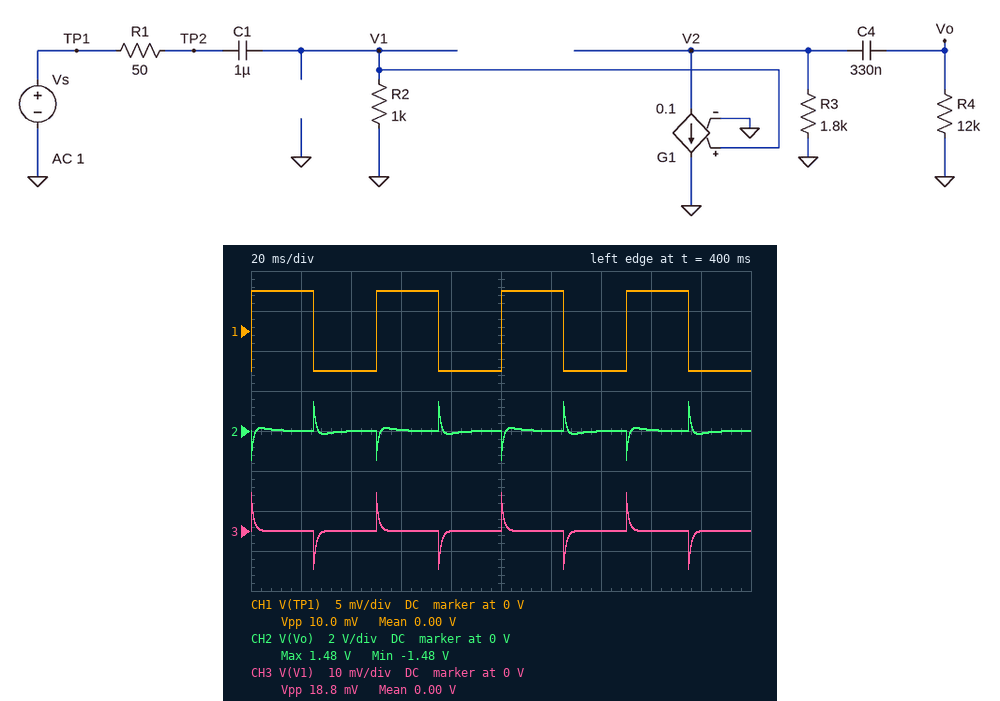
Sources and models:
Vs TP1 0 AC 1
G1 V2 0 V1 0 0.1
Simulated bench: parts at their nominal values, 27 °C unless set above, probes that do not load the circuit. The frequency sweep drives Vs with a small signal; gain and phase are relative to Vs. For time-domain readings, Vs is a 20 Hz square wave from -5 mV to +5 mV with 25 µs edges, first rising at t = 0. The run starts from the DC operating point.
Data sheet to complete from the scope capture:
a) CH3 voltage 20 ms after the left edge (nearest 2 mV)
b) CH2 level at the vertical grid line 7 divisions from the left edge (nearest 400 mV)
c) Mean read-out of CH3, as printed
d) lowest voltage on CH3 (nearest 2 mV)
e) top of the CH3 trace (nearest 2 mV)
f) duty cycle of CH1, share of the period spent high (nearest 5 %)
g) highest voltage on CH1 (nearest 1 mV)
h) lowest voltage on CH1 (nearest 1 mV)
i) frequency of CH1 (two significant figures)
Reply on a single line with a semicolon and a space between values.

0 V; 0 V; 0.00 V; -10 mV; 10 mV; 50 %; 5 mV; -5 mV; 20 Hz
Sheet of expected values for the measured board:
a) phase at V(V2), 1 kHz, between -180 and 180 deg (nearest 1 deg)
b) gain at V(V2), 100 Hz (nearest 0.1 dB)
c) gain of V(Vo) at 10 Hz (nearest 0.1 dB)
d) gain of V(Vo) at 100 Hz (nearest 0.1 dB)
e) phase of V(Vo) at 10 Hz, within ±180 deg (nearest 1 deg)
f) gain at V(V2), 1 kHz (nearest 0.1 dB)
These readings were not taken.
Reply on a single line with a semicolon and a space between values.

-172 deg; 38.4 dB; 8.6 dB; 37.8 dB; -20 deg; 43.4 dB
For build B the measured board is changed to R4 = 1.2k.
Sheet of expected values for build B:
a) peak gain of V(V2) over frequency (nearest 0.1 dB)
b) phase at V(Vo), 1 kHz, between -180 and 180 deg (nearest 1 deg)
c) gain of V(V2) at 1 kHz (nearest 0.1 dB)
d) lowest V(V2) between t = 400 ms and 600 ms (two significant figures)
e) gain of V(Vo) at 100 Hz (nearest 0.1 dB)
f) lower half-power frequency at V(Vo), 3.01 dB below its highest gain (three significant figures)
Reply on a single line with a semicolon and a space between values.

39.6 dB; -162 deg; 37.2 dB; -750 mV; 26.0 dB; 243 Hz
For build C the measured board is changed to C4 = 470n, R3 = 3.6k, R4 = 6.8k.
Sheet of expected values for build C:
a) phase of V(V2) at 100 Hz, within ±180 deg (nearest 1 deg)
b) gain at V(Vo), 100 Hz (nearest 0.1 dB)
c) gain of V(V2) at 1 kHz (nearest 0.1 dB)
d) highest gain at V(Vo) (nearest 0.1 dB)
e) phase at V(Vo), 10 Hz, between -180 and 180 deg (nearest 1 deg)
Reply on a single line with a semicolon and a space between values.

-132 deg; 41.4 dB; 46.9 dB; 47.0 dB; -21 deg
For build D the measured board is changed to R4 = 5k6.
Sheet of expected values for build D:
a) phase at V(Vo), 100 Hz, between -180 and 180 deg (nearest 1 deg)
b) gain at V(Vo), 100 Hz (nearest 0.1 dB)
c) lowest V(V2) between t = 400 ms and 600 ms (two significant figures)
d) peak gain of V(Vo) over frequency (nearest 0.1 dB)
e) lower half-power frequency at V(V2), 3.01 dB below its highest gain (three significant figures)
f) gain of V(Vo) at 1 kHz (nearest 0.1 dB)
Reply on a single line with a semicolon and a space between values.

-90 deg; 35.5 dB; -1.3 V; 42.3 dB; 134 Hz; 42.1 dB
